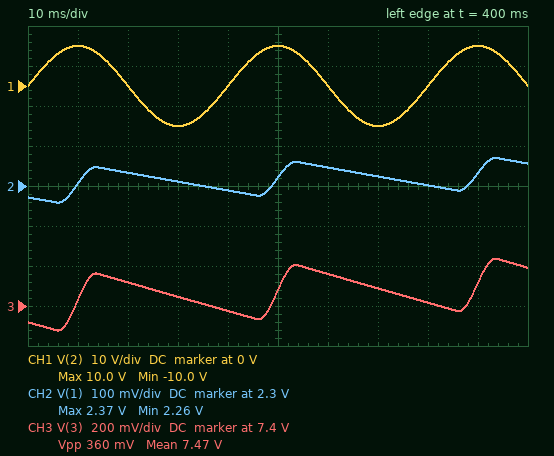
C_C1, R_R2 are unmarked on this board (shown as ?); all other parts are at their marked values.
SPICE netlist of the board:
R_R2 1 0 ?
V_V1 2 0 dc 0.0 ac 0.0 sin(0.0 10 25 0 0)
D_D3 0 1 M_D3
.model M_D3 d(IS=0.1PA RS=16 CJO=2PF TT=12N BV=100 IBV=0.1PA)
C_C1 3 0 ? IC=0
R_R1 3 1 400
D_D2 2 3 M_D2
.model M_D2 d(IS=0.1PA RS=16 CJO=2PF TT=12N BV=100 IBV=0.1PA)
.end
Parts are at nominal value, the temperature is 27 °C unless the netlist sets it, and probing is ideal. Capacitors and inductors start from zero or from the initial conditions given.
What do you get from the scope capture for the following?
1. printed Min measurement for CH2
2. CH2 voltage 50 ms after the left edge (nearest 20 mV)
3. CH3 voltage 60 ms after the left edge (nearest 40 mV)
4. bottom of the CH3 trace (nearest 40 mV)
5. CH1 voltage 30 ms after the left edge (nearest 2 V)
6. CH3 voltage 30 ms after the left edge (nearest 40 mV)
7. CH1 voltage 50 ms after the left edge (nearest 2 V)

2.26 V
2.32 V
7.56 V
7.28 V
-10 V
7.44 V
10 V
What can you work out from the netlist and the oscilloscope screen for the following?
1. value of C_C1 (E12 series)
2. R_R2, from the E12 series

1.8 mF
180 Ω
